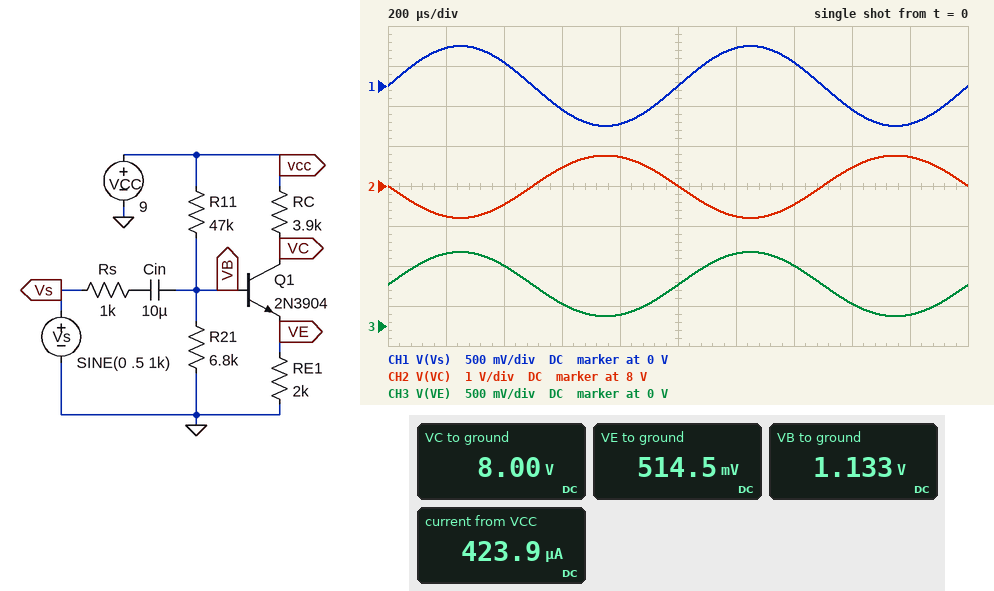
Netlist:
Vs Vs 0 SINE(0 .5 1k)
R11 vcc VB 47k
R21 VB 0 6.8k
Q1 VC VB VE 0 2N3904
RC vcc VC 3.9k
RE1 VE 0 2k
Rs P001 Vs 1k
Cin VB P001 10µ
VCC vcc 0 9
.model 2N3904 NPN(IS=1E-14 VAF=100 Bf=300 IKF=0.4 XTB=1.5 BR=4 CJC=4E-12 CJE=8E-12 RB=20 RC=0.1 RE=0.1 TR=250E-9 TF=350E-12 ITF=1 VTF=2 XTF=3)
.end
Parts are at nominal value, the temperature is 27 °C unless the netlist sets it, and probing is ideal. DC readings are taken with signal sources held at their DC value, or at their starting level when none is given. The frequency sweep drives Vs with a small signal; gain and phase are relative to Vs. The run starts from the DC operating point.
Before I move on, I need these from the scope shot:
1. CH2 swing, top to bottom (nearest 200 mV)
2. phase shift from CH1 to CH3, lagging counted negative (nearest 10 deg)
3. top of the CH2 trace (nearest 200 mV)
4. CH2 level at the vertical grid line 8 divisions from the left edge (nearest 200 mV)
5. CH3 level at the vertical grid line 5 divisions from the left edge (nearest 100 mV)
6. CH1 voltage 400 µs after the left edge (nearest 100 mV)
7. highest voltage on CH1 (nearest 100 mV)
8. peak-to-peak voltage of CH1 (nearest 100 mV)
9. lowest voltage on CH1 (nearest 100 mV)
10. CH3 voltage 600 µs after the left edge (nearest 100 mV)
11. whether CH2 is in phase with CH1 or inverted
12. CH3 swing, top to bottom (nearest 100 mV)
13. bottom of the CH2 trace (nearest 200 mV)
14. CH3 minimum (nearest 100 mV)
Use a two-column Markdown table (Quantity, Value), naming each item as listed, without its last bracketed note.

| Quantity | Value |
|---|---|
| CH2 swing, top to bottom | 1.6 V |
| phase shift from CH1 to CH3, lagging counted negative | 0 deg |
| top of the CH2 trace | 8.8 V |
| CH2 level at the vertical grid line 8 divisions from the left edge | 8.4 V |
| CH3 level at the vertical grid line 5 divisions from the left edge | 500 mV |
| CH1 voltage 400 µs after the left edge | 300 mV |
| highest voltage on CH1 | 500 mV |
| peak-to-peak voltage of CH1 | 1.0 V |
| lowest voltage on CH1 | -500 mV |
| CH3 voltage 600 µs after the left edge | 300 mV |
| whether CH2 is in phase with CH1 or inverted | inverted |
| CH3 swing, top to bottom | 800 mV |
| bottom of the CH2 trace | 7.2 V |
| CH3 minimum | 100 mV |
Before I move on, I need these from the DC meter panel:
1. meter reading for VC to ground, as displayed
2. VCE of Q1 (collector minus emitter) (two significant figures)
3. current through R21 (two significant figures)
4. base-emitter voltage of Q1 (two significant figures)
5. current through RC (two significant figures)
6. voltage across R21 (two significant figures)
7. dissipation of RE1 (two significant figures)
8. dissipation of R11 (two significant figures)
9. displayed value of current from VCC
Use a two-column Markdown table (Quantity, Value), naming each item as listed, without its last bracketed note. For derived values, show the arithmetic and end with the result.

| Quantity | Value |
|---|---|
| meter reading for VC to ground, as displayed | 8.00 V |
| VCE of Q1 (collector minus emitter) | 8 V - 514.5 mV = 7.5 V |
| current through R21 | (1.133 V) / 6.8 kΩ = 170 µA |
| base-emitter voltage of Q1 | 1.133 V - 514.5 mV = 620 mV |
| current through RC | (9 V - 8 V) / 3.9 kΩ = 260 µA |
| voltage across R21 | 1.133 V = 1.1 V |
| dissipation of RE1 | (514.5 mV)^2 / 2 kΩ = 130 µW |
| dissipation of R11 | (9 V - 1.133 V)^2 / 47 kΩ = 1.3 mW |
| displayed value of current from VCC | 423.9 µA |
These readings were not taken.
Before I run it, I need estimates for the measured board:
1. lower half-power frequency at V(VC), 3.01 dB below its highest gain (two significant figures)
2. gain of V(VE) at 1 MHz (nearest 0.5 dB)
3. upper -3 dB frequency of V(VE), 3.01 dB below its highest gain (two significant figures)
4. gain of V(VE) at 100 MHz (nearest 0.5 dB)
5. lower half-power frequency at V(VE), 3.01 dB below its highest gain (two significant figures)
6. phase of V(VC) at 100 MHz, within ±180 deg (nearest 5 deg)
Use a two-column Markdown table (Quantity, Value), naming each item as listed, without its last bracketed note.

| Quantity | Value |
|---|---|
| lower half-power frequency at V(VC), 3.01 dB below its highest gain | 2.3 Hz |
| gain of V(VE) at 1 MHz | -2.0 dB |
| upper -3 dB frequency of V(VE), 3.01 dB below its highest gain | 22 MHz |
| gain of V(VE) at 100 MHz | -6.0 dB |
| lower half-power frequency at V(VE), 3.01 dB below its highest gain | 2.3 Hz |
| phase of V(VC) at 100 MHz, within ±180 deg | 20 deg |
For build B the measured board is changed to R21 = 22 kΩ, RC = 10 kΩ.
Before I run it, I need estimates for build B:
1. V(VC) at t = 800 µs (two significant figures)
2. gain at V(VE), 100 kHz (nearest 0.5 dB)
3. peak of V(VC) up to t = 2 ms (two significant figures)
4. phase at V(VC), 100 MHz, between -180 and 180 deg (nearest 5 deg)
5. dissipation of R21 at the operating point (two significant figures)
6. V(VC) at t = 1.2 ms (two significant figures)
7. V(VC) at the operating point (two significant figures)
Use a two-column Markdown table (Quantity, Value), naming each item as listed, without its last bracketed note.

| Quantity | Value |
|---|---|
| V(VC) at t = 800 µs | 3.2 V |
| gain at V(VE), 100 kHz | -4.5 dB |
| peak of V(VC) up to t = 2 ms | 3.3 V |
| phase at V(VC), 100 MHz, between -180 and 180 deg | 0 deg |
| dissipation of R21 at the operating point | 220 µW |
| V(VC) at t = 1.2 ms | 1.9 V |
| V(VC) at the operating point | 1.6 V |
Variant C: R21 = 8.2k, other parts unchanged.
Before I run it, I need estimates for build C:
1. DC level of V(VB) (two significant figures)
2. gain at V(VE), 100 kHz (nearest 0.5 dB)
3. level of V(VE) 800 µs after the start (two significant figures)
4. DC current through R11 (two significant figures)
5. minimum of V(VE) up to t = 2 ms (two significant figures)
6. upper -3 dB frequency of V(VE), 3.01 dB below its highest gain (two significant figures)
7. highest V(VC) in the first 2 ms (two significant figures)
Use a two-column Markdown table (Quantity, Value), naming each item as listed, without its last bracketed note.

| Quantity | Value |
|---|---|
| DC level of V(VB) | 1.3 V |
| gain at V(VE), 100 kHz | -1.5 dB |
| level of V(VE) 800 µs after the start | 310 mV |
| DC current through R11 | 160 µA |
| minimum of V(VE) up to t = 2 ms | 290 mV |
| upper -3 dB frequency of V(VE), 3.01 dB below its highest gain | 21 MHz |
| highest V(VC) in the first 2 ms | 8.4 V |
